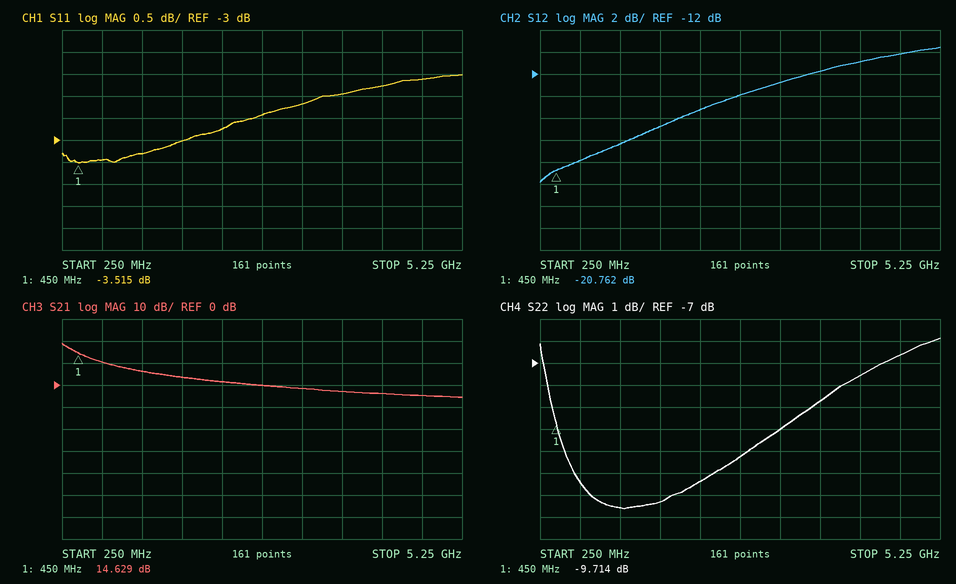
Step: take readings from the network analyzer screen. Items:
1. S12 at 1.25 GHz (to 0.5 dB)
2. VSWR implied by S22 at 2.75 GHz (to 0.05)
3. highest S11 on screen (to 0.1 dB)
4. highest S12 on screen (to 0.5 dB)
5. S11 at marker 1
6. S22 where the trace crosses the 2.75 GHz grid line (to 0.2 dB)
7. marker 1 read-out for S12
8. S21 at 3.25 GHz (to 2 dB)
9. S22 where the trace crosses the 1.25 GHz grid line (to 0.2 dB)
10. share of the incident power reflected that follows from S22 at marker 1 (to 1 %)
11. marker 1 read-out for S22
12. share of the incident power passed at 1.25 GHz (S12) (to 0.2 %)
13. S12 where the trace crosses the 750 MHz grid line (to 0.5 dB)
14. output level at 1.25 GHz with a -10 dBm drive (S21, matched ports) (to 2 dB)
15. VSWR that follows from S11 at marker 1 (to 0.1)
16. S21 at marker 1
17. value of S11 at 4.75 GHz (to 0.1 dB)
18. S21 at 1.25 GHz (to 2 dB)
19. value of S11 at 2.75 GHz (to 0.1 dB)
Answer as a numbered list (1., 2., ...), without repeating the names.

1. -18.5 dB
2. 1.75
3. -1.5 dB
4. -9.5 dB
5. -3.515 dB
6. -11.2 dB
7. -20.762 dB
8. -2 dB
9. -13.6 dB
10. 11 %
11. -9.714 dB
12. 1.4 %
13. -20.0 dB
14. -4 dBm
15. 5.0
16. 14.629 dB
17. -1.6 dB
18. 6 dB
19. -2.4 dB
